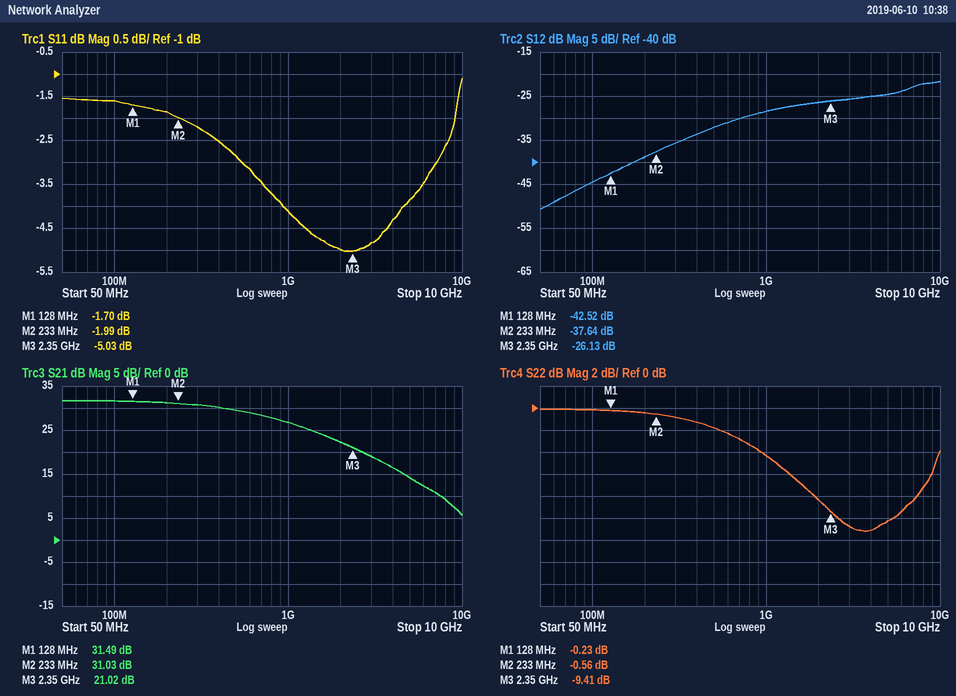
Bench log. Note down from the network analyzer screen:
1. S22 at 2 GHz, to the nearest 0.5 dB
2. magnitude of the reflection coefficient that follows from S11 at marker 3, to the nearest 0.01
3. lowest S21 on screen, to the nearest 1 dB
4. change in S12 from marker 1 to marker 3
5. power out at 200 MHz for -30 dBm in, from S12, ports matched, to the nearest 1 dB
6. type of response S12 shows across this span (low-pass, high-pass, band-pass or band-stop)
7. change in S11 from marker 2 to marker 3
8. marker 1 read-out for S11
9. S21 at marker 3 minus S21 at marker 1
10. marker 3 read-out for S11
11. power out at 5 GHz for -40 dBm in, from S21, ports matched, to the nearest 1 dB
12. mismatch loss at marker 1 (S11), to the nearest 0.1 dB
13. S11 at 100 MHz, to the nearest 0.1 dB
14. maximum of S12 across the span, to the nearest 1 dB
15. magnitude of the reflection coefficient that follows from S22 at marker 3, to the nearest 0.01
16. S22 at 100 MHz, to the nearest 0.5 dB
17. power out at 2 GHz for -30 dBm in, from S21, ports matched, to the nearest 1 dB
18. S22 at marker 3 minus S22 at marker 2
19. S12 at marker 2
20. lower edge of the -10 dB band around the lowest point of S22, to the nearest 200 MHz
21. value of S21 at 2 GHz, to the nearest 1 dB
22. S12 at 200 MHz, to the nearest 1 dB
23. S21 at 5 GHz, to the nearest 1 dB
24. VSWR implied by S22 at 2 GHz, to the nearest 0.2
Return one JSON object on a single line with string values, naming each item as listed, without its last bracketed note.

{"S22 at 2 GHz, to the nearest 0.5 dB": "-8.5 dB", "magnitude of the reflection coefficient that follows from S11 at marker 3, to the nearest 0.01": "0.56", "lowest S21 on screen, to the nearest 1 dB": "6 dB", "change in S12 from marker 1 to marker 3": "16.39 dB", "power out at 200 MHz for -30 dBm in, from S12, ports matched, to the nearest 1 dB": "-69 dBm", "type of response S12 shows across this span": "high-pass", "change in S11 from marker 2 to marker 3": "-3.04 dB", "marker 1 read-out for S11": "-1.70 dB", "S21 at marker 3 minus S21 at marker 1": "-10.47 dB", "marker 3 read-out for S11": "-5.03 dB", "power out at 5 GHz for -40 dBm in, from S21, ports matched, to the nearest 1 dB": "-26 dBm", "mismatch loss at marker 1 (S11), to the nearest 0.1 dB": "4.9 dB", "S11 at 100 MHz, to the nearest 0.1 dB": "-1.6 dB", "maximum of S12 across the span, to the nearest 1 dB": "-22 dB", "magnitude of the reflection coefficient that follows from S22 at marker 3, to the nearest 0.01": "0.34", "S22 at 100 MHz, to the nearest 0.5 dB": "0.0 dB", "power out at 2 GHz for -30 dBm in, from S21, ports matched, to the nearest 1 dB": "-8 dBm", "S22 at marker 3 minus S22 at marker 2": "-8.85 dB", "S12 at marker 2": "-37.64 dB", "lower edge of the -10 dB band around the lowest point of S22, to the nearest 200 MHz": "2.6 GHz", "value of S21 at 2 GHz, to the nearest 1 dB": "22 dB", "S12 at 200 MHz, to the nearest 1 dB": "-39 dB", "S21 at 5 GHz, to the nearest 1 dB": "14 dB", "VSWR implied by S22 at 2 GHz, to the nearest 0.2": "2.2"}
